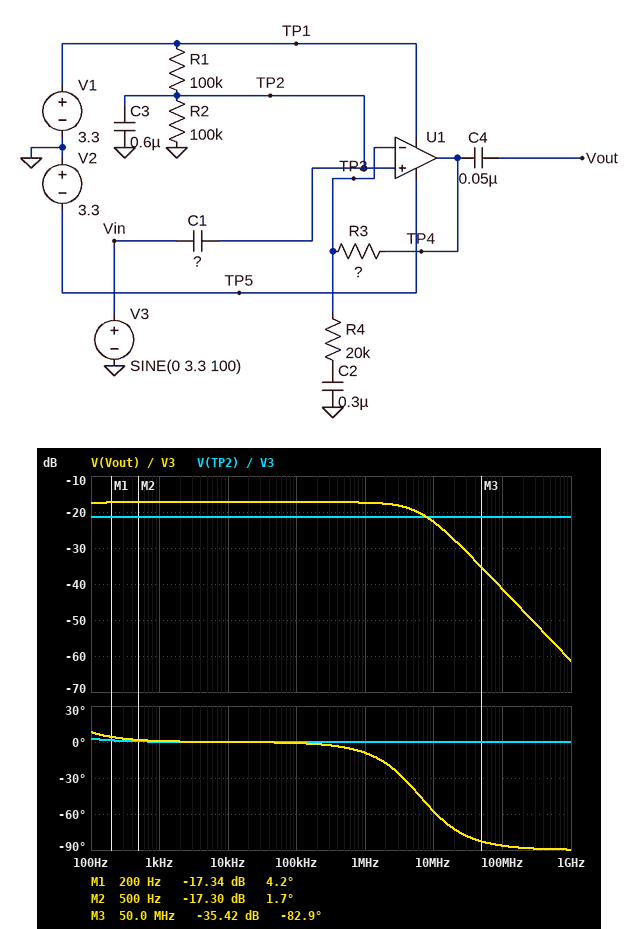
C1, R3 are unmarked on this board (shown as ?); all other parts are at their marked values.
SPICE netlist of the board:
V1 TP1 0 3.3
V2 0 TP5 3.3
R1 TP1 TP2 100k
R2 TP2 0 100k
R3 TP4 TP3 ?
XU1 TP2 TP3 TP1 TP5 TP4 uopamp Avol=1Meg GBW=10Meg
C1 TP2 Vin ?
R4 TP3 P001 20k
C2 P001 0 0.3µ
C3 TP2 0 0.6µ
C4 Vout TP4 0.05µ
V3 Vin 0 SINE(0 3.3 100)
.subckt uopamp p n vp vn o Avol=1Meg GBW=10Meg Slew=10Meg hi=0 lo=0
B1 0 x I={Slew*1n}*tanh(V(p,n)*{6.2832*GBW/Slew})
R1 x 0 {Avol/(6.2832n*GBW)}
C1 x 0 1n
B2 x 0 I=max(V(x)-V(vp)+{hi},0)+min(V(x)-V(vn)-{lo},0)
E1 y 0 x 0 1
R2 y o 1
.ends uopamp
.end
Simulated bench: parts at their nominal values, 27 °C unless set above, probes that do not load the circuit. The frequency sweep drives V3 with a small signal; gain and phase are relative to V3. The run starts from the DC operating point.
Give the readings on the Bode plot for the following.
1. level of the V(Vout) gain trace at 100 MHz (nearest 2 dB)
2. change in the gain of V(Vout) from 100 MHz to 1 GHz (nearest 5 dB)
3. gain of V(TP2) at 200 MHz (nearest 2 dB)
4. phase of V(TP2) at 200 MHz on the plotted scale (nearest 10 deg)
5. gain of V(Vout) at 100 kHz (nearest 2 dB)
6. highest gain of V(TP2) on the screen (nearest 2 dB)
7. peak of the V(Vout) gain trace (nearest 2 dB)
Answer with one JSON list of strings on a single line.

["-42 dB", "-20 dB", "-22 dB", "0 deg", "-18 dB", "-22 dB", "-18 dB"]
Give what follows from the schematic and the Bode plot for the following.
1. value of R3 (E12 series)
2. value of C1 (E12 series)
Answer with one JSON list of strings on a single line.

["12 kΩ", "56 nF"]
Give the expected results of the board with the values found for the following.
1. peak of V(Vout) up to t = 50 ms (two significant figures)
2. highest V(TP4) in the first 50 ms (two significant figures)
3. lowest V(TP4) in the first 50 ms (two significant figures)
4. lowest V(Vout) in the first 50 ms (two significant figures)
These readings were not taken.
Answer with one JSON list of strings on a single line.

["440 mV", "2.1 V", "1.2 V", "-470 mV"]
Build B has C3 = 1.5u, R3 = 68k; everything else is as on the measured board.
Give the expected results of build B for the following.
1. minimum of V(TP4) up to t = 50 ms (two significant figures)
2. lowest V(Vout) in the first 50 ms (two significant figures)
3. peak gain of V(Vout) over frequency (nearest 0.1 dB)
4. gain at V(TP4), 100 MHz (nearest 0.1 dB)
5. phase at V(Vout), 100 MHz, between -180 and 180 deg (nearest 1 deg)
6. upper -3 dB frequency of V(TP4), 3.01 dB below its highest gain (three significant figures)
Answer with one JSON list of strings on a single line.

["1.1 V", "-540 mV", "-16.0 dB", "-48.9 dB", "-89 deg", "2.27 MHz"]
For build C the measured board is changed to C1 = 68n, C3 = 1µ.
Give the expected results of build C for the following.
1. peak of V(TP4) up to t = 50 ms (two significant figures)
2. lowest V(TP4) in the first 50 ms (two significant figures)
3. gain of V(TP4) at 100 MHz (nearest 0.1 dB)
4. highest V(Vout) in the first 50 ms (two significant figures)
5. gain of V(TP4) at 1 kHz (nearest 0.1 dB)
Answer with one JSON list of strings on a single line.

["2.0 V", "1.3 V", "-43.9 dB", "330 mV", "-19.8 dB"]
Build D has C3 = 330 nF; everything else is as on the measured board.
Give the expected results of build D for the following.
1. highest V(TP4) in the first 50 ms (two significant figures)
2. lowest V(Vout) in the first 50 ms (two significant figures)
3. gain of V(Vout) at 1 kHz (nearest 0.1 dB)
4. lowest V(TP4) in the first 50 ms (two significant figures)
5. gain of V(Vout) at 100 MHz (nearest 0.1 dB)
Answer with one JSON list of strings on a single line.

["2.4 V", "-800 mV", "-12.7 dB", "850 mV", "-36.8 dB"]
